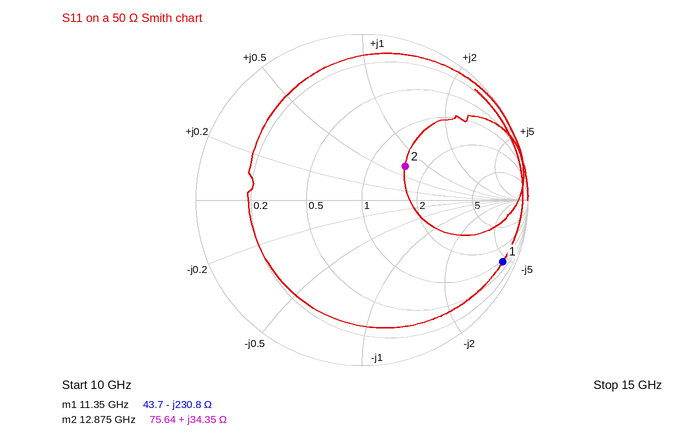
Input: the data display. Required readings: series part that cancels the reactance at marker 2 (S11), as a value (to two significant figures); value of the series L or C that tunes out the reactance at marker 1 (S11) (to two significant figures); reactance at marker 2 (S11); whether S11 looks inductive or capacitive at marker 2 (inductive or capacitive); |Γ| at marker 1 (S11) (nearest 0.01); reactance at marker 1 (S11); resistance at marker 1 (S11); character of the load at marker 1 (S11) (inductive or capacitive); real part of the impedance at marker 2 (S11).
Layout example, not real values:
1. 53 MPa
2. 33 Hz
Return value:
1. 360 fF
2. 3.2 nH
3. +34.35 Ω
4. inductive
5. 0.93
6. -230.8 Ω
7. 43.7 Ω
8. capacitive
9. 75.64 Ω
